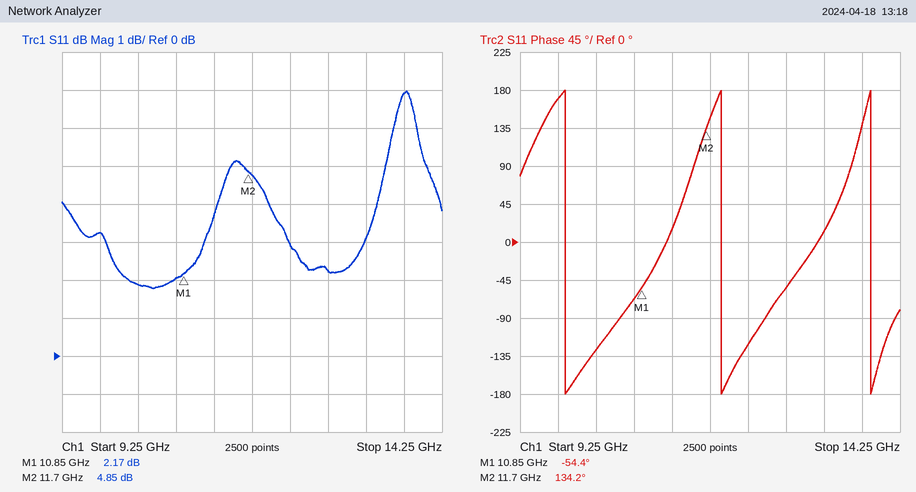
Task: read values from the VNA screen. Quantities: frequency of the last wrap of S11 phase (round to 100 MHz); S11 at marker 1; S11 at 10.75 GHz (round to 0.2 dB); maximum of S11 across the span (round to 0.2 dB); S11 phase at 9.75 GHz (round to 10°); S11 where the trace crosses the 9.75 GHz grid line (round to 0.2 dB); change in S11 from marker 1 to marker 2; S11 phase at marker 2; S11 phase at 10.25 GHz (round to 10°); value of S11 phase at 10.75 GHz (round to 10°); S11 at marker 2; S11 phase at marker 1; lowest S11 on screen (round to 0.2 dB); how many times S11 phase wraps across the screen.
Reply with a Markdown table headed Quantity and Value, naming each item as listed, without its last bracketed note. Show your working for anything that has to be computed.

| Quantity | Value |
|---|---|
| frequency of the last wrap of S11 phase | 13.9 GHz |
| S11 at marker 1 | 2.17 dB |
| S11 at 10.75 GHz | 2.0 dB |
| maximum of S11 across the span | 7.0 dB |
| S11 phase at 9.75 GHz | 170° |
| S11 where the trace crosses the 9.75 GHz grid line | 3.2 dB |
| change in S11 from marker 1 to marker 2 | 4.85 − (2.17) = 2.68 dB |
| S11 phase at marker 2 | 134.2° |
| S11 phase at 10.25 GHz | -130° |
| value of S11 phase at 10.75 GHz | -70° |
| S11 at marker 2 | 4.85 dB |
| S11 phase at marker 1 | -54.4° |
| lowest S11 on screen | 1.8 dB |
| how many times S11 phase wraps across the screen | 3 |
